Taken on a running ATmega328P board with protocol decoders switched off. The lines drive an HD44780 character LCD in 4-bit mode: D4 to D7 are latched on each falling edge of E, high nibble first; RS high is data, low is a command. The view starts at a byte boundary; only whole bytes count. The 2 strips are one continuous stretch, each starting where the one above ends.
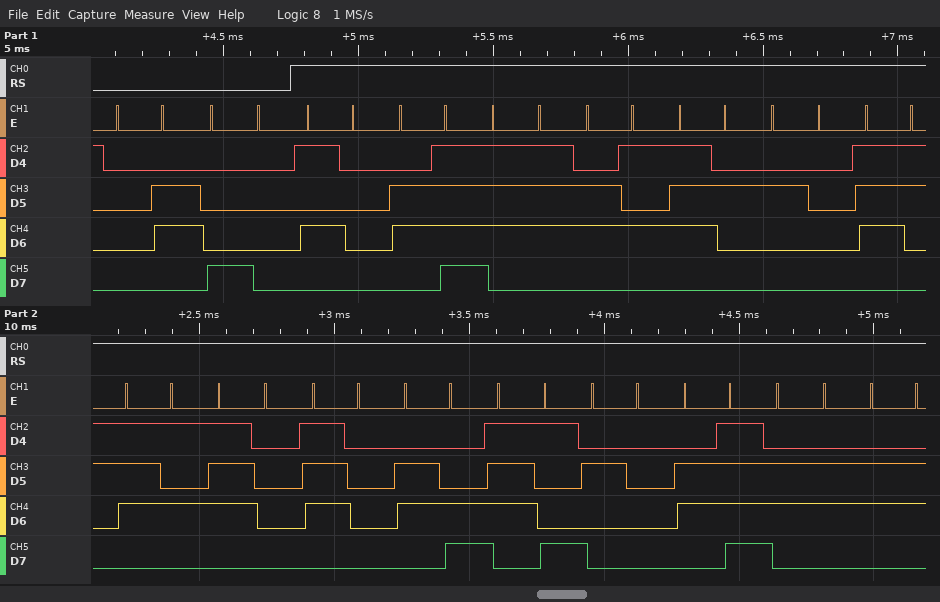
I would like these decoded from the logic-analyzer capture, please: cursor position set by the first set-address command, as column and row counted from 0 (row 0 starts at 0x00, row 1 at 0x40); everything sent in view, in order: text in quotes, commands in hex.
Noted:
column 0, row 0
0x06 0x80 "Power supply off"
